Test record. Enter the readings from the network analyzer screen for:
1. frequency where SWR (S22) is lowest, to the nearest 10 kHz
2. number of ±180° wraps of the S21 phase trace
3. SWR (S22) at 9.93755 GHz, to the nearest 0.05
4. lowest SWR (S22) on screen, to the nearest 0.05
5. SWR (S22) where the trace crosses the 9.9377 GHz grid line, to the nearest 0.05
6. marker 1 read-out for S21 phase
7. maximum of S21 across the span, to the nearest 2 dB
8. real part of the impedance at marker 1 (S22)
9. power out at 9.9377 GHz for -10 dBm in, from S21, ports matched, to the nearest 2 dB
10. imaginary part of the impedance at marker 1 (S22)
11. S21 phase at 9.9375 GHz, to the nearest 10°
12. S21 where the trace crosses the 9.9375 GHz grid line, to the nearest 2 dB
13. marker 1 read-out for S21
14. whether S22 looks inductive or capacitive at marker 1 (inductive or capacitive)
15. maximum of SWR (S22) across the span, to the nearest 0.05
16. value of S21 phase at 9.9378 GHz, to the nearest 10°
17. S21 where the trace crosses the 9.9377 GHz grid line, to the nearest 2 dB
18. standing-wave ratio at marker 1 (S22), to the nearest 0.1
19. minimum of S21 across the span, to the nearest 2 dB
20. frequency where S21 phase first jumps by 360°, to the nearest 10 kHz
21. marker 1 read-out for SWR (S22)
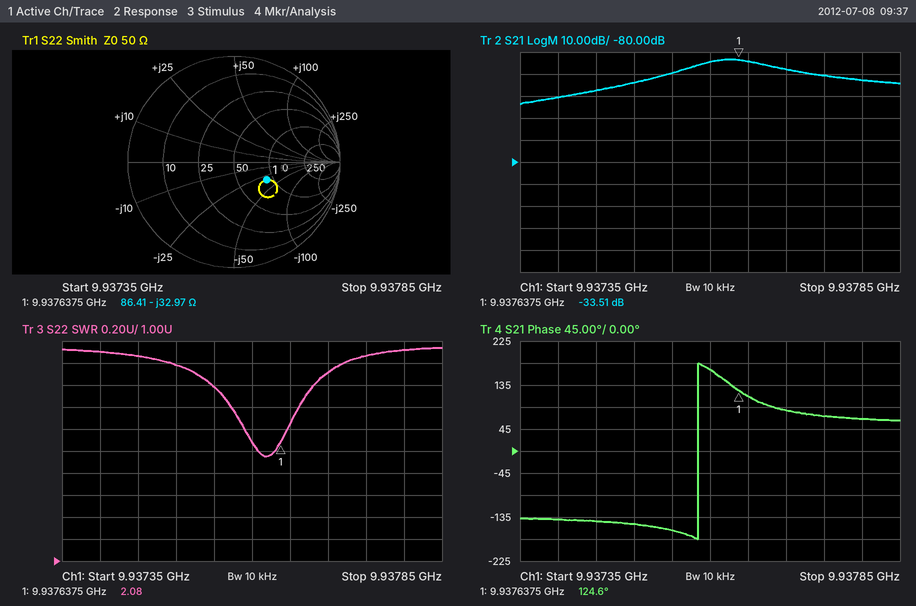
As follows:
9.93762 GHz
1
2.60
1.95
2.70
124.6°
-34 dB
86.41 Ω
-48 dBm
-32.97 Ω
-150°
-44 dB
-33.51 dB
capacitive
2.95
70°
-38 dB
2.1
-54 dB
9.93758 GHz
2.08
